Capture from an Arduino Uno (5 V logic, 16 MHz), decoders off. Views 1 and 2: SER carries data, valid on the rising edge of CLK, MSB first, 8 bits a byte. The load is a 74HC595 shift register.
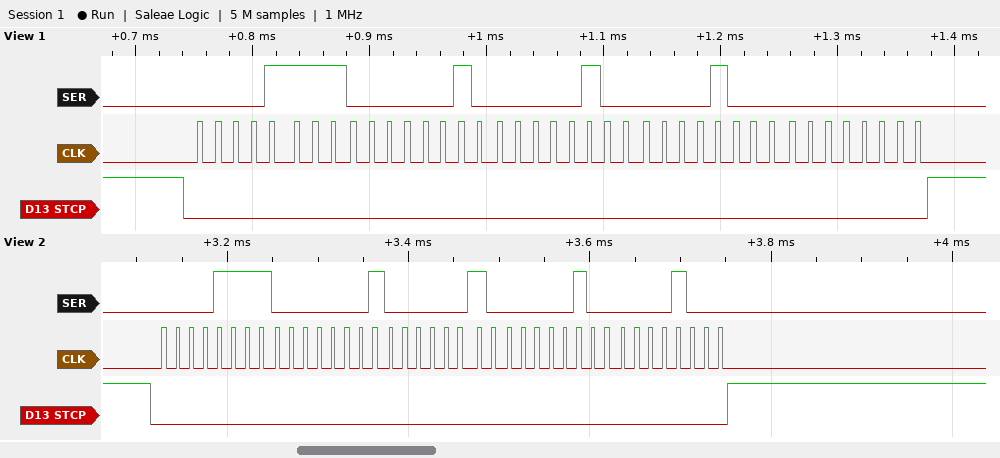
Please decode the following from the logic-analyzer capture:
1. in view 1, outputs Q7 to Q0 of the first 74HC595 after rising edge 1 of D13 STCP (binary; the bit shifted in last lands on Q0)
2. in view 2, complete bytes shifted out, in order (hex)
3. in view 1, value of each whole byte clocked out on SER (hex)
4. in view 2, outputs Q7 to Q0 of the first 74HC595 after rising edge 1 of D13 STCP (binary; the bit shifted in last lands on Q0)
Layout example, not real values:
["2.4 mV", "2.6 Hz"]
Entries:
["00000000", "0F 01 02 04 08", "0x0F 0x02 0x04 0x08 0x00", "00001000"]
